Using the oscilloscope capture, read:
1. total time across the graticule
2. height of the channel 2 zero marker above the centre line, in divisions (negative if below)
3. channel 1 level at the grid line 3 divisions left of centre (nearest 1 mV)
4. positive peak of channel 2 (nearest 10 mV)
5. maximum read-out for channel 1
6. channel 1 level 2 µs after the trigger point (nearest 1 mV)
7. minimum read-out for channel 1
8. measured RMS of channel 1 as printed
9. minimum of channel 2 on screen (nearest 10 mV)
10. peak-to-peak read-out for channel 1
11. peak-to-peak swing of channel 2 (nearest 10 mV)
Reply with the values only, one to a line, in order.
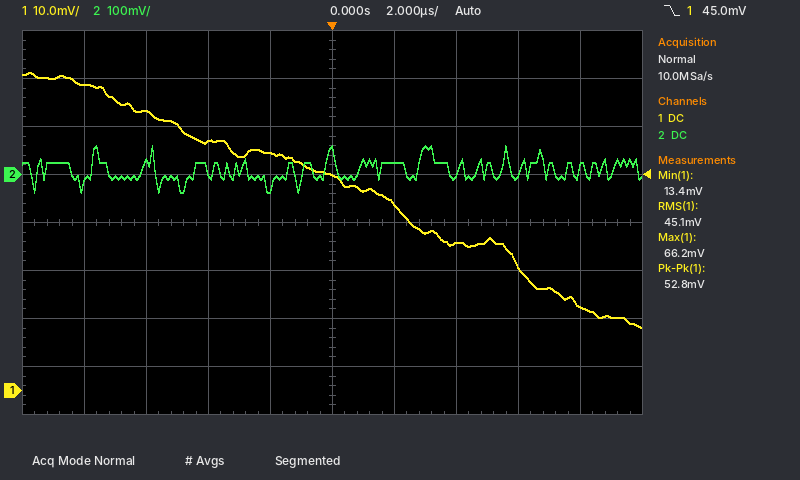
20 µs
+1.0 div
58 mV
60 mV
66.2 mV
39 mV
13.4 mV
45.1 mV
-40 mV
52.8 mV
100 mV
